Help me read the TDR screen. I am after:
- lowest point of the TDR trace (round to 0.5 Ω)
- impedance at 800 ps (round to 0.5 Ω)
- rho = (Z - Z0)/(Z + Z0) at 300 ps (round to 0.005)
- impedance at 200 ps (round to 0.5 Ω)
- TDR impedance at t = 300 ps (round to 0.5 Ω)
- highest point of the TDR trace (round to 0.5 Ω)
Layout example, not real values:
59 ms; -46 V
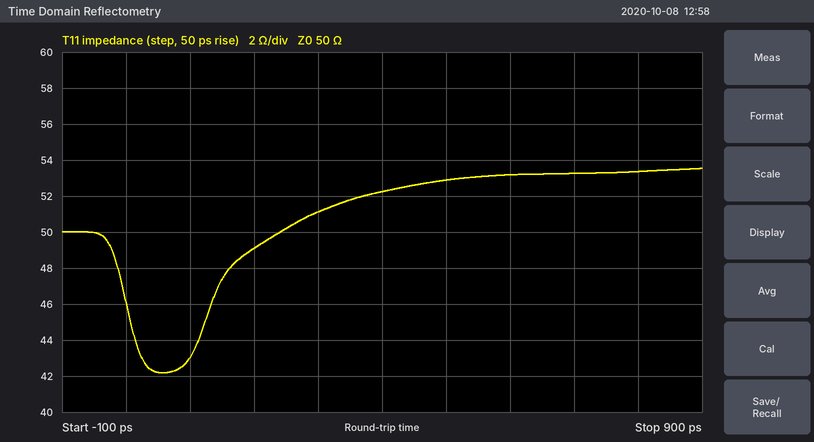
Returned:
42.0 Ω; 53.5 Ω; +0.010; 49.0 Ω; 51.0 Ω; 53.5 Ω
